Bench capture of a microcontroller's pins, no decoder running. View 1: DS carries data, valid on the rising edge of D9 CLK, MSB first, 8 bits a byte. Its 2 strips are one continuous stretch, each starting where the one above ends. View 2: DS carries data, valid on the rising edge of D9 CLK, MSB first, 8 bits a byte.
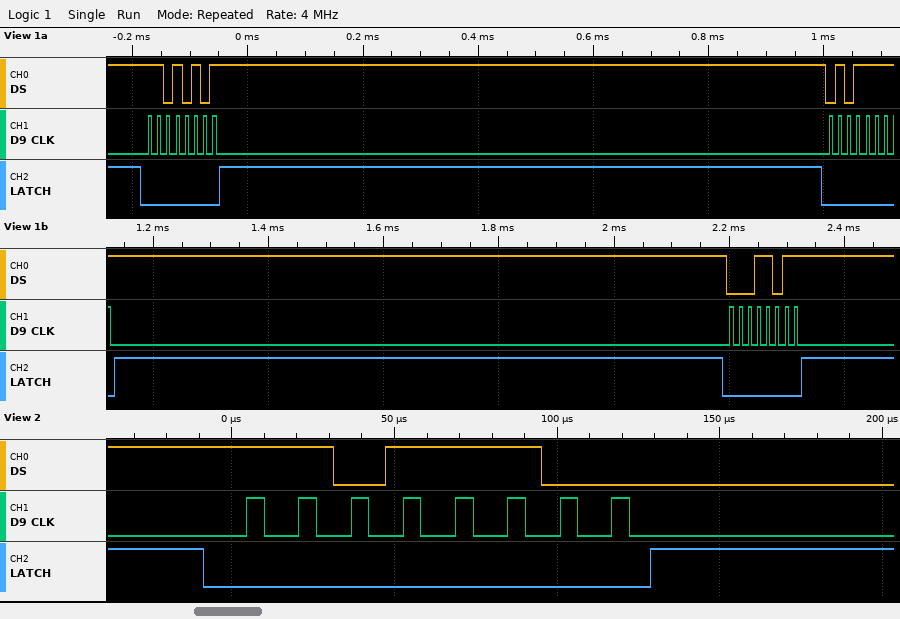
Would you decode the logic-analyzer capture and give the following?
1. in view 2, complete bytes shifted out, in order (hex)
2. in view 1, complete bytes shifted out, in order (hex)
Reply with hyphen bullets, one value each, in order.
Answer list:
- DC
- 0xD5 0x5F 0x1B
